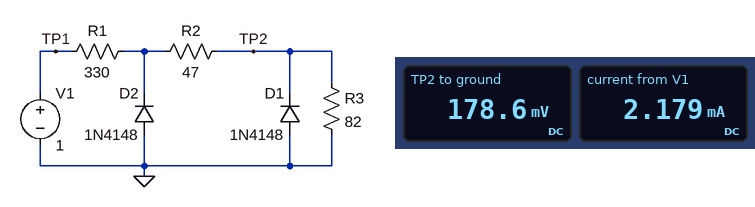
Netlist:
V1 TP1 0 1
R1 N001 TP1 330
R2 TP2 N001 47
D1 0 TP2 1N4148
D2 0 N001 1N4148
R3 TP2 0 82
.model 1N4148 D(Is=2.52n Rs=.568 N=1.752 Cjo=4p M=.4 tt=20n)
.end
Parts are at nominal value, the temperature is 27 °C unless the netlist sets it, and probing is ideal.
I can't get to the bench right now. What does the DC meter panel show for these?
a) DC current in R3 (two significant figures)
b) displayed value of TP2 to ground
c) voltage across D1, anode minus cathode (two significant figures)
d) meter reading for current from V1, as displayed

2.2 mA
178.6 mV
-180 mV
2.179 mA
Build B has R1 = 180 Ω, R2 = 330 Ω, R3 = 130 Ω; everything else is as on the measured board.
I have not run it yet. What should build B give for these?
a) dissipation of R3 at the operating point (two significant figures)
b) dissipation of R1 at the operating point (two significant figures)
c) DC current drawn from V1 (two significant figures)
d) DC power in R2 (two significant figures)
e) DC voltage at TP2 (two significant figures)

320 µW
440 µW
1.6 mA
810 µW
200 mV
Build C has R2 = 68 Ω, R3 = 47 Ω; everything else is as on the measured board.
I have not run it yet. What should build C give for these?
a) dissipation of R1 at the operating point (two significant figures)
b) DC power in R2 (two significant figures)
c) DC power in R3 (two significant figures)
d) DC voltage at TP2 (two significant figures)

1.7 mW
340 µW
240 µW
110 mV
